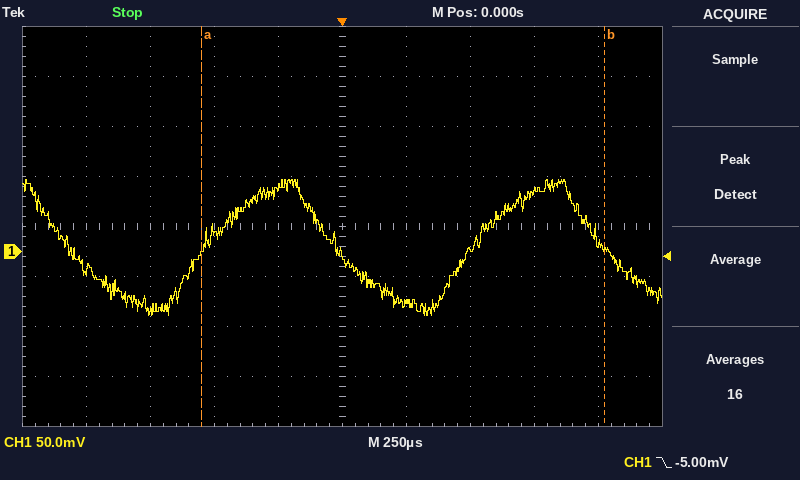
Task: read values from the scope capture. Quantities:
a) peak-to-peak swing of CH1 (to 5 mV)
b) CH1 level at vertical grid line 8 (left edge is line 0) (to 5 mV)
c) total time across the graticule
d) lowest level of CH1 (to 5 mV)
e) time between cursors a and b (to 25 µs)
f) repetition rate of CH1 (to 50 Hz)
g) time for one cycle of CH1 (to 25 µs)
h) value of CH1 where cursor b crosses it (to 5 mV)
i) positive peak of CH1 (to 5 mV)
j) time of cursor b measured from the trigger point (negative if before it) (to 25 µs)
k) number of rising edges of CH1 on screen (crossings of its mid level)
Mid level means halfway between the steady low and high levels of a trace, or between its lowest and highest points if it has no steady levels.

135 mV
60 mV
2.5 ms
-65 mV
1.575 ms
950 Hz
1.050 ms
5 mV
70 mV
+1.025 ms
2
